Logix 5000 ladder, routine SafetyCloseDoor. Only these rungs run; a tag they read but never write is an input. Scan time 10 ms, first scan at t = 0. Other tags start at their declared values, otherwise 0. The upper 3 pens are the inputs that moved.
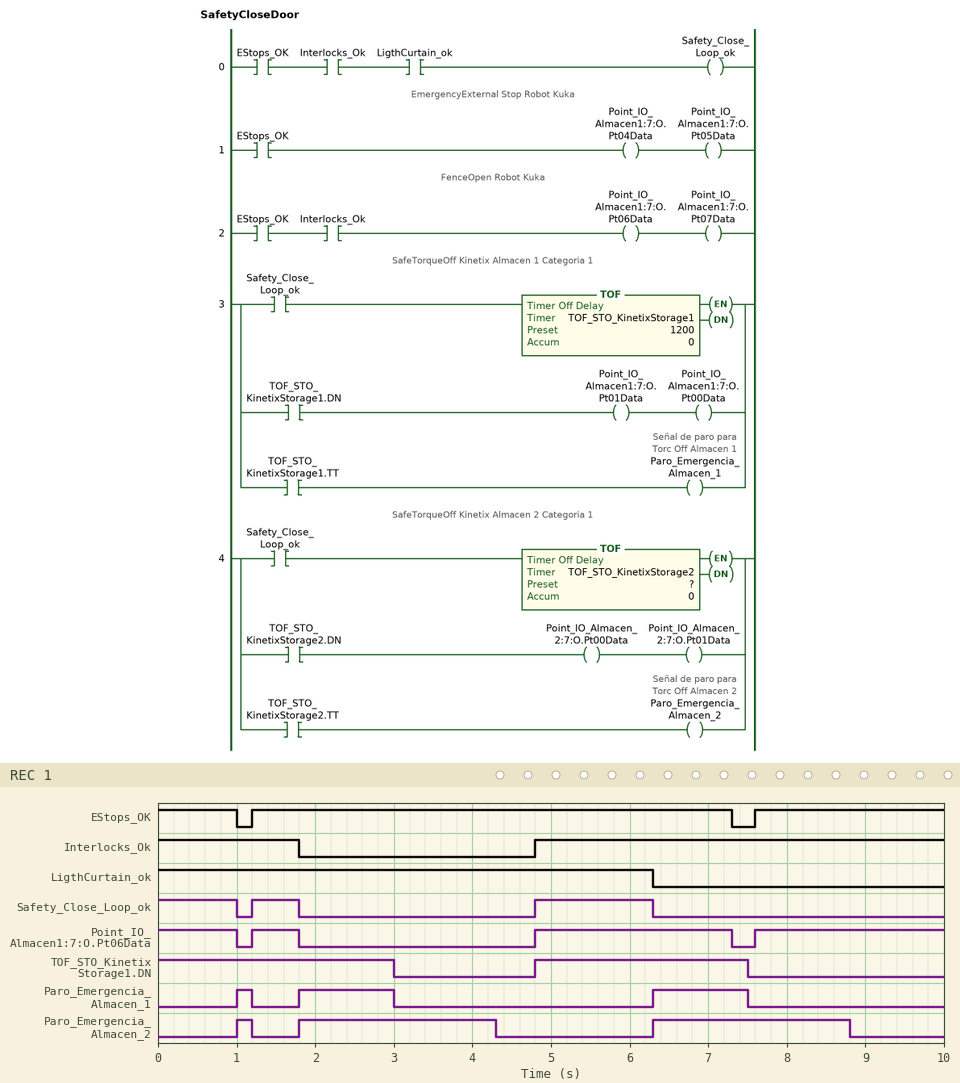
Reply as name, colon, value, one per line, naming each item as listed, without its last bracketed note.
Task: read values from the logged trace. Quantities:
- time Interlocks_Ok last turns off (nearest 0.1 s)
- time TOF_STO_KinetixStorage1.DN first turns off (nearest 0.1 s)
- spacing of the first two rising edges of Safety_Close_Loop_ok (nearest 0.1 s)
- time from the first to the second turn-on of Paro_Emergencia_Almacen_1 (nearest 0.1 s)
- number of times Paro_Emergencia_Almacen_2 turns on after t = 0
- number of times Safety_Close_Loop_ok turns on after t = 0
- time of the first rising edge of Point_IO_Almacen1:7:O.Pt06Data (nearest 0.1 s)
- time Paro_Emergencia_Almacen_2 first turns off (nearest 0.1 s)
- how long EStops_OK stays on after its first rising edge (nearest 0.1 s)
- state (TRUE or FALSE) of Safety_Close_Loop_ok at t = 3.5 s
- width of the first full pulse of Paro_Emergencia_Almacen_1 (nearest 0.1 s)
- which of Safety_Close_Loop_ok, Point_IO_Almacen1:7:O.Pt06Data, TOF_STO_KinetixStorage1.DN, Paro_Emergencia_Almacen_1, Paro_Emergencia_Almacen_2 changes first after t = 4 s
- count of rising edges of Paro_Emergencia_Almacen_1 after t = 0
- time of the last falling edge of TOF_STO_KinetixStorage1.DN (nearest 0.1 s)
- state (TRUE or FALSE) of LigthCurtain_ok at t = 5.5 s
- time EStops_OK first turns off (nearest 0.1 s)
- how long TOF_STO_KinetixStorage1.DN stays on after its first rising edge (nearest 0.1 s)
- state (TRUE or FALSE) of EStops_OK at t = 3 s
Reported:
time Interlocks_Ok last turns off: 1.8 s
time TOF_STO_KinetixStorage1.DN first turns off: 3.0 s
spacing of the first two rising edges of Safety_Close_Loop_ok: 3.6 s
time from the first to the second turn-on of Paro_Emergencia_Almacen_1: 0.8 s
number of times Paro_Emergencia_Almacen_2 turns on after t = 0: 3
number of times Safety_Close_Loop_ok turns on after t = 0: 2
time of the first rising edge of Point_IO_Almacen1:7:O.Pt06Data: 1.2 s
time Paro_Emergencia_Almacen_2 first turns off: 1.2 s
how long EStops_OK stays on after its first rising edge: 6.1 s
state (TRUE or FALSE) of Safety_Close_Loop_ok at t = 3.5 s: FALSE
width of the first full pulse of Paro_Emergencia_Almacen_1: 0.2 s
which of Safety_Close_Loop_ok, Point_IO_Almacen1:7:O.Pt06Data, TOF_STO_KinetixStorage1.DN, Paro_Emergencia_Almacen_1, Paro_Emergencia_Almacen_2 changes first after t = 4 s: Paro_Emergencia_Almacen_2
count of rising edges of Paro_Emergencia_Almacen_1 after t = 0: 3
time of the last falling edge of TOF_STO_KinetixStorage1.DN: 7.5 s
state (TRUE or FALSE) of LigthCurtain_ok at t = 5.5 s: TRUE
time EStops_OK first turns off: 1.0 s
how long TOF_STO_KinetixStorage1.DN stays on after its first rising edge: 2.7 s
state (TRUE or FALSE) of EStops_OK at t = 3 s: TRUE
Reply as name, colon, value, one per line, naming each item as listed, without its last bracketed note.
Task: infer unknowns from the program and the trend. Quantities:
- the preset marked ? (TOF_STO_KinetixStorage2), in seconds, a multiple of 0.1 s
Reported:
the preset marked ? (TOF_STO_KinetixStorage2), in seconds, a multiple of 0.1 s: 2.5 s
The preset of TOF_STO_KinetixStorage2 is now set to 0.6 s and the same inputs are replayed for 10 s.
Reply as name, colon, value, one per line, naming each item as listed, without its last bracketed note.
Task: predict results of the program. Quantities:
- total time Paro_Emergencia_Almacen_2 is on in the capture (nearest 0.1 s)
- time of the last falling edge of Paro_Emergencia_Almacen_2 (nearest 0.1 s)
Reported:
total time Paro_Emergencia_Almacen_2 is on in the capture: 1.4 s
time of the last falling edge of Paro_Emergencia_Almacen_2: 6.9 s
